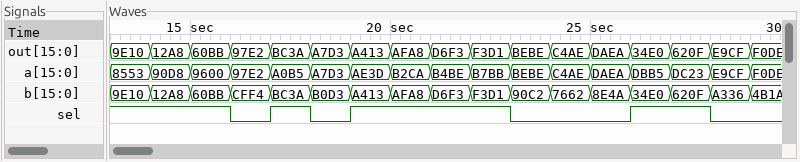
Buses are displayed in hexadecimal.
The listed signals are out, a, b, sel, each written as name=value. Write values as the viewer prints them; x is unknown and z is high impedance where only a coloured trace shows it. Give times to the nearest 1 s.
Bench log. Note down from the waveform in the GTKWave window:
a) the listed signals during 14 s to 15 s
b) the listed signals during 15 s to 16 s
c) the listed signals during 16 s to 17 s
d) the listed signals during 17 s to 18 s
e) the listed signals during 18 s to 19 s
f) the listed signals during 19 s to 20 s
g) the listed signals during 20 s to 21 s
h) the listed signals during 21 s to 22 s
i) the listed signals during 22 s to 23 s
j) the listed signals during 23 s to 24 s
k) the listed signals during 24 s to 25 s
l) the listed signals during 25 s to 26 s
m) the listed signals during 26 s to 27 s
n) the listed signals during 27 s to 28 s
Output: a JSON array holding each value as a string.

["out=12A8, a=90D8, b=12A8, sel=1", "out=60BB, a=9600, b=60BB, sel=1", "out=97E2, a=97E2, b=CFF4, sel=0", "out=BC3A, a=A0B5, b=BC3A, sel=1", "out=A7D3, a=A7D3, b=B0D3, sel=0", "out=A413, a=AE3D, b=A413, sel=1", "out=AFA8, a=B2CA, b=AFA8, sel=1", "out=D6F3, a=B4BE, b=D6F3, sel=1", "out=F3D1, a=B7BB, b=F3D1, sel=1", "out=BEBE, a=BEBE, b=90C2, sel=0", "out=C4AE, a=C4AE, b=7662, sel=0", "out=DAEA, a=DAEA, b=8E4A, sel=0", "out=34E0, a=DBB5, b=34E0, sel=1", "out=620F, a=DC23, b=620F, sel=1"]
